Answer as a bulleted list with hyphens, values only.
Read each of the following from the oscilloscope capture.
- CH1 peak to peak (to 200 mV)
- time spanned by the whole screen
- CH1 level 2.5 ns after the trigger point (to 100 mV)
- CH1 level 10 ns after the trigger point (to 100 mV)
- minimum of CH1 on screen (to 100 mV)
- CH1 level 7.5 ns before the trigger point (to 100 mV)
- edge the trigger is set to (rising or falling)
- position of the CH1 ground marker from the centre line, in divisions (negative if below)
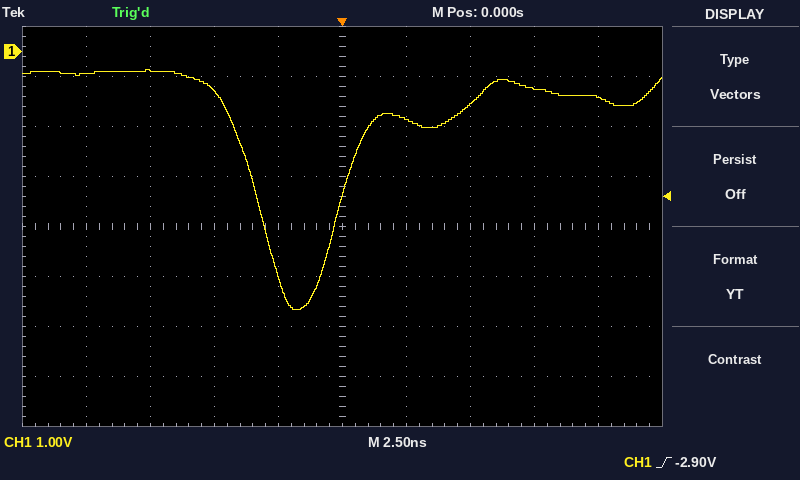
- 4.8 V
- 25 ns
- -1.4 V
- -900 mV
- -5.2 V
- -400 mV
- rising
- +3.5 div
